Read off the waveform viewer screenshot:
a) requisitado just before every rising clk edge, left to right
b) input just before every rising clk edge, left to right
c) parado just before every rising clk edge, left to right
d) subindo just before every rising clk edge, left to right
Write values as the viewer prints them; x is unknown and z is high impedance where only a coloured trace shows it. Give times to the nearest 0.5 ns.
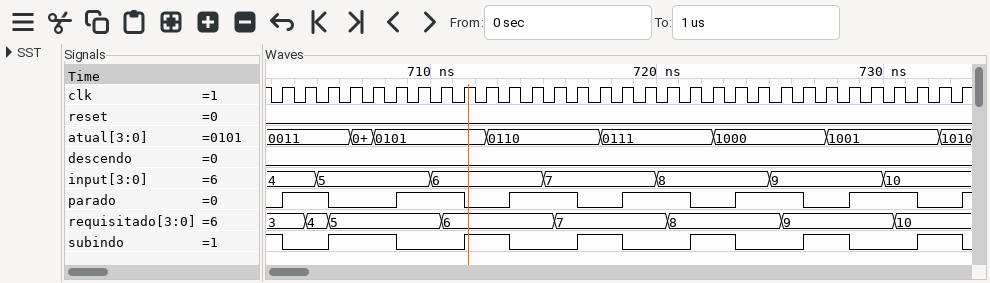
3, 3, 4, 5, 5, 5, 5, 5, 6, 6, 6, 6, 6, 7, 7, 7, 7, 7, 8, 8, 8, 8, 8, 9, 9, 9, 9, 9, 10, 10, 10
4, 4, 5, 5, 5, 5, 5, 6, 6, 6, 6, 6, 7, 7, 7, 7, 7, 8, 8, 8, 8, 8, 9, 9, 9, 9, 9, 10, 10, 10, 10
0 1 1 0 0 0 1 1 1 0 0 1 1 1 0 0 1 1 1 0 0 1 1 1 0 0 1 1 1 0 0
1 0 0 1 1 1 0 0 0 1 1 0 0 0 1 1 0 0 0 1 1 0 0 0 1 1 0 0 0 1 1
